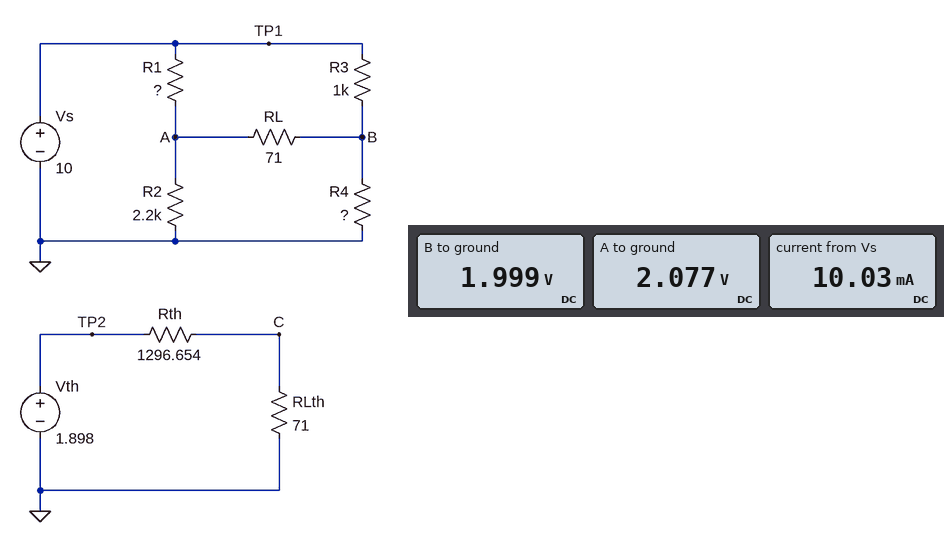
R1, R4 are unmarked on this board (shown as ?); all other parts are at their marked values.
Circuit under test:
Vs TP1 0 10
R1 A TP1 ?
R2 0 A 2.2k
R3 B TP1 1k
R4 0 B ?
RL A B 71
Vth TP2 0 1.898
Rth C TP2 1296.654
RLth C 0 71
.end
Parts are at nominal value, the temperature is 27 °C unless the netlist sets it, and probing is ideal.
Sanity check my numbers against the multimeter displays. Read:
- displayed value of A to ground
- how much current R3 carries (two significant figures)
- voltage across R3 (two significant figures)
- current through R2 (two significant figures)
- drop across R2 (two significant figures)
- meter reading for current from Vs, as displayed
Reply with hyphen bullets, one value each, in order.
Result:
- 2.077 V
- 8.0 mA
- 8.0 V
- 940 µA
- 2.1 V
- 10.03 mA
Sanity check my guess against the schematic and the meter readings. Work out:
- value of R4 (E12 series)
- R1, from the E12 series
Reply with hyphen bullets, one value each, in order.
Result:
- 220 Ω
- 3.9 kΩ
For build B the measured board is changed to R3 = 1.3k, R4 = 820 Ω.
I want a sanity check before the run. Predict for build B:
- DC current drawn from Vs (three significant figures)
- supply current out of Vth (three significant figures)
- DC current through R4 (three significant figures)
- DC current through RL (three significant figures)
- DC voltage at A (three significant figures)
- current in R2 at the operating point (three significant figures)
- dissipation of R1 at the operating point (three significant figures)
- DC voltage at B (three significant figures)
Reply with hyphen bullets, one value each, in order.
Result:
- 6.36 mA
- 1.39 mA
- 4.64 mA
- 132 µA
- 3.79 V
- 1.72 mA
- 9.88 mW
- 3.80 V
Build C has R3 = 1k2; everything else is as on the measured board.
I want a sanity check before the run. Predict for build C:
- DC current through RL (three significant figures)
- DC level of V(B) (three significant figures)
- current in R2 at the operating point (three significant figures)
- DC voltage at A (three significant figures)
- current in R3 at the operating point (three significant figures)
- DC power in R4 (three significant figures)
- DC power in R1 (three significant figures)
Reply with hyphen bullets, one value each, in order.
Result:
- 1.24 mA
- 1.78 V
- 849 µA
- 1.87 V
- 6.85 mA
- 14.4 mW
- 17.0 mW
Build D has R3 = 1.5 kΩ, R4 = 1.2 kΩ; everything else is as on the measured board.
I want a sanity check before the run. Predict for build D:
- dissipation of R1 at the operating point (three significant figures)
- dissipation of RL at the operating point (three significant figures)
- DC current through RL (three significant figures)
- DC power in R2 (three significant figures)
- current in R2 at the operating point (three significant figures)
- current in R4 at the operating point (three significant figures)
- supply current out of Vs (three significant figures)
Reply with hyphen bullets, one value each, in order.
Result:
- 8.76 mW
- 10.8 µW
- 391 µA
- 7.85 mW
- 1.89 mA
- 3.49 mA
- 5.38 mA
